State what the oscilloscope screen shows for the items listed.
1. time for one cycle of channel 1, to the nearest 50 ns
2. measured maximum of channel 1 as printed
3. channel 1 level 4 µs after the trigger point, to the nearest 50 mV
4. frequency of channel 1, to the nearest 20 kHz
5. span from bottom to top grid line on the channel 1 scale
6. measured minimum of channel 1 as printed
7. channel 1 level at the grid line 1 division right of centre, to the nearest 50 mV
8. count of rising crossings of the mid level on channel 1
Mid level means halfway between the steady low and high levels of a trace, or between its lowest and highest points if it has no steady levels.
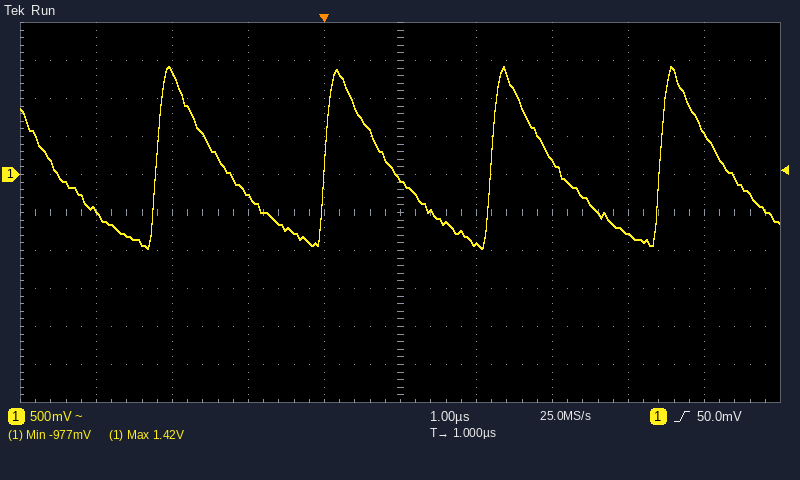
2.20 µs
1.42 V
-800 mV
460 kHz
5 V
-977 mV
-900 mV
4
